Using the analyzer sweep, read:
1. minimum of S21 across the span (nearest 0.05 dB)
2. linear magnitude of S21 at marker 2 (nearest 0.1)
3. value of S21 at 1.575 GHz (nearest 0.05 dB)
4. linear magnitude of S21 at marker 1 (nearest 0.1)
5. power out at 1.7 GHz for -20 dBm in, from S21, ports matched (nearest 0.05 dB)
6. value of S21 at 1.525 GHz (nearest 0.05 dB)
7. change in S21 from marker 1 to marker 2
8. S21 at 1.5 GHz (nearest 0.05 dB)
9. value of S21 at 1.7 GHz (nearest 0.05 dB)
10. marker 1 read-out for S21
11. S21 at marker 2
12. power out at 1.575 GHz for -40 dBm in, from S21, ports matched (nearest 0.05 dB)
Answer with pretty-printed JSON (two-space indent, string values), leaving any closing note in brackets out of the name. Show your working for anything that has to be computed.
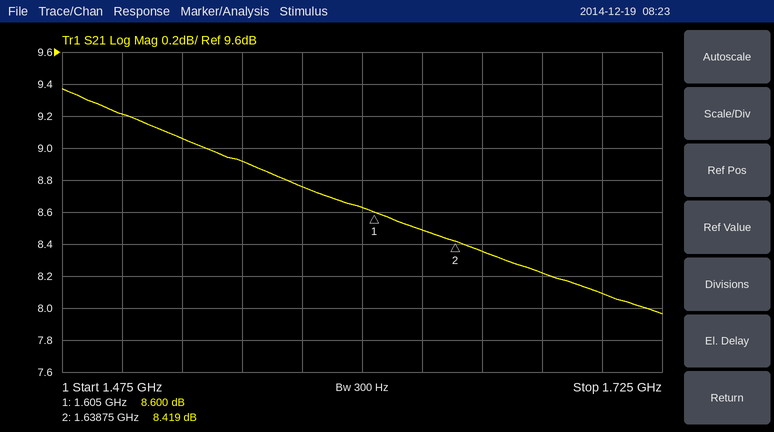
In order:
{
  "minimum of S21 across the span": "7.95 dB",
  "linear magnitude of S21 at marker 2": "10^(8.419/20) ≈ 2.6",
  "value of S21 at 1.575 GHz": "8.75 dB",
  "linear magnitude of S21 at marker 1": "10^(8.6/20) ≈ 2.7",
  "power out at 1.7 GHz for -20 dBm in, from S21, ports matched": "-20 dBm + (8.10 dB) = -11.90 dBm",
  "value of S21 at 1.525 GHz": "9.05 dB",
  "change in S21 from marker 1 to marker 2": "8.419 − (8.6) = -0.181 dB",
  "S21 at 1.5 GHz": "9.20 dB",
  "value of S21 at 1.7 GHz": "8.10 dB",
  "marker 1 read-out for S21": "8.600 dB",
  "S21 at marker 2": "8.419 dB",
  "power out at 1.575 GHz for -40 dBm in, from S21, ports matched": "-40 dBm + (8.75 dB) = -31.25 dBm"
}
